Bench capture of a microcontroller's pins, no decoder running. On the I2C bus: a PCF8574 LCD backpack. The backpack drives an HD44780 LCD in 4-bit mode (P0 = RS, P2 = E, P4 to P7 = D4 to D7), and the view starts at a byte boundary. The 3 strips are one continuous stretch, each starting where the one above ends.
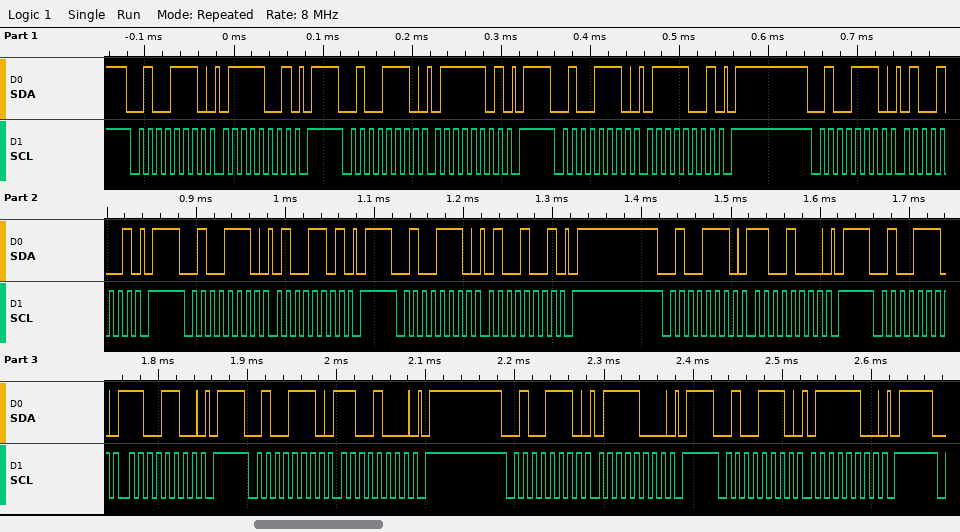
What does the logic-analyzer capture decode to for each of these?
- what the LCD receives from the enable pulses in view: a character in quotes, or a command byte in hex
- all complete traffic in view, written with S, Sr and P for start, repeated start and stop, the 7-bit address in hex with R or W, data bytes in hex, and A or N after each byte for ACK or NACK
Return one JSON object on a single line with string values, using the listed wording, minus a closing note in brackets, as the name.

{"what the LCD receives from the enable pulses in view: a character in quotes, or a command byte in hex": "'t'", "all complete traffic in view, written with S, Sr and P for start, repeated start and stop, the 7-bit address in hex with R or W, data bytes in hex, and A or N after each byte for ACK or NACK": "S 27W A 79 A P S 27W A 7D A P S 27W A 79 A P S 27W A 49 A P S 27W A 4D A P S 27W A 49 A P S 27W A C8 A P S 27W A CC A P S 27W A C8 A P S 27W A 78 A P S 27W A 7C A P"}
